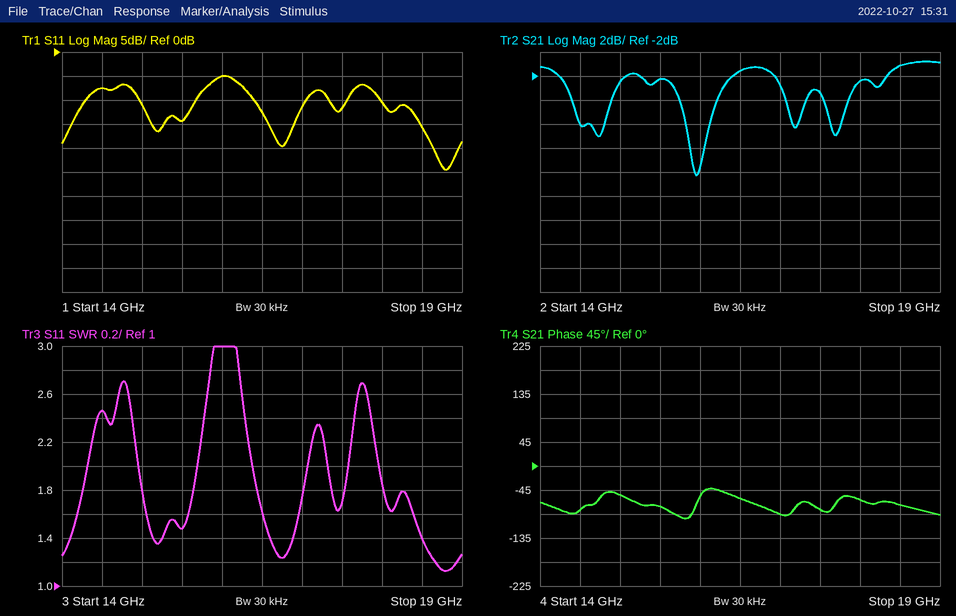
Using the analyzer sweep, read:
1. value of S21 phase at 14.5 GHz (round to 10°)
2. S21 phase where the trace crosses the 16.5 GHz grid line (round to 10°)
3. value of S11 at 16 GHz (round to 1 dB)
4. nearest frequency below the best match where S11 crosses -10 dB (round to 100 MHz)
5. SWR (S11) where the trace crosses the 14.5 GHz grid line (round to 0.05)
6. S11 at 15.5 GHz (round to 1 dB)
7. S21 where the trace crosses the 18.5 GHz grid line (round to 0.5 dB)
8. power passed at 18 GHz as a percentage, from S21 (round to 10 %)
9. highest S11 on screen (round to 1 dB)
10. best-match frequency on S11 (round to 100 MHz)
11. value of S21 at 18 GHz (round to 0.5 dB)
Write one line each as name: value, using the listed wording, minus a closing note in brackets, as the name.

value of S21 phase at 14.5 GHz: -80°
S21 phase where the trace crosses the 16.5 GHz grid line: -60°
value of S11 at 16 GHz: -5 dB
nearest frequency below the best match where S11 crosses -10 dB: 18.0 GHz
SWR (S11) where the trace crosses the 14.5 GHz grid line: 2.45
S11 at 15.5 GHz: -14 dB
S21 where the trace crosses the 18.5 GHz grid line: -1.0 dB
power passed at 18 GHz as a percentage, from S21: 60 %
highest S11 on screen: -5 dB
best-match frequency on S11: 18.8 GHz
value of S21 at 18 GHz: -2.5 dB
